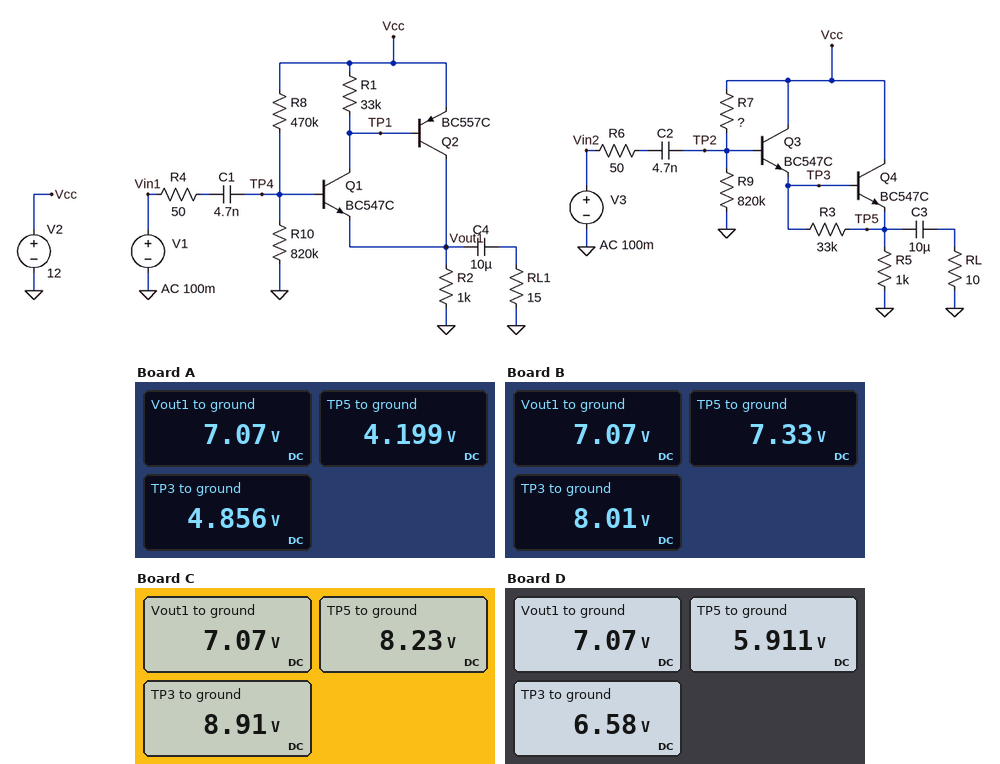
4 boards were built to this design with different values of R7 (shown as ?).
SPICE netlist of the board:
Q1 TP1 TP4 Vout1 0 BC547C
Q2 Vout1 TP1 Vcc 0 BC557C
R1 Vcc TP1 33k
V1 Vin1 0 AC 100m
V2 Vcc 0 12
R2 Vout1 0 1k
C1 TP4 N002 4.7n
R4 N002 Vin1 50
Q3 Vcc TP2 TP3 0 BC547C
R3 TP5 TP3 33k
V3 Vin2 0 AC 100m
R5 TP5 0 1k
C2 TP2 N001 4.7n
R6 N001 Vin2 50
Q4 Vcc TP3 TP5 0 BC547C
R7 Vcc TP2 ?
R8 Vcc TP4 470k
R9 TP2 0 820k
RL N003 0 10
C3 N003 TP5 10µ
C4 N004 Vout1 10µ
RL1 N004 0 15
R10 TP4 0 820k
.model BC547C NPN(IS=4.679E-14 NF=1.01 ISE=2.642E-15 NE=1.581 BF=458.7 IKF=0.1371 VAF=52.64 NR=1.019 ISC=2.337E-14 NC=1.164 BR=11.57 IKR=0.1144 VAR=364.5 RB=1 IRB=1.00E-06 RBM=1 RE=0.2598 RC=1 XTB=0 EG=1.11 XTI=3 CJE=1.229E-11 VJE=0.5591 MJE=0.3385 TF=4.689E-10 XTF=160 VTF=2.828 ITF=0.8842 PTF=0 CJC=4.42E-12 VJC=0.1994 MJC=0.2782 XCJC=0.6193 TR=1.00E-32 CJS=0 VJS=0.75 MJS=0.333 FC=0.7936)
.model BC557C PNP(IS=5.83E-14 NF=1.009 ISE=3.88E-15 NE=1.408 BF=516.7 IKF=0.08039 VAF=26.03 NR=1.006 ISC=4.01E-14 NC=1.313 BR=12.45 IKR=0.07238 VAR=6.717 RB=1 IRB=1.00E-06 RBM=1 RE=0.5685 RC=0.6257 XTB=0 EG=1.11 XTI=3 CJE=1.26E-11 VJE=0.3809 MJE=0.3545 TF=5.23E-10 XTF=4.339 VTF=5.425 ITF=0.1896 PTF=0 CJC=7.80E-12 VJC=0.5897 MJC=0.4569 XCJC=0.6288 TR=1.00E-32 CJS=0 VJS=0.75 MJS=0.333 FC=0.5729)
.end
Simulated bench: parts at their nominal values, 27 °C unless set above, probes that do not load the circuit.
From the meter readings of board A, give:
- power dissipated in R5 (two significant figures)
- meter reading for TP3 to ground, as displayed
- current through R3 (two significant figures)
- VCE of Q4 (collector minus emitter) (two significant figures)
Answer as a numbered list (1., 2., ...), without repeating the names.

1. 18 mW
2. 4.856 V
3. 20 µA
4. 7.8 V
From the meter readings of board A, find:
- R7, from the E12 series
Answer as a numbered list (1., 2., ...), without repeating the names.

1. 1 MΩ
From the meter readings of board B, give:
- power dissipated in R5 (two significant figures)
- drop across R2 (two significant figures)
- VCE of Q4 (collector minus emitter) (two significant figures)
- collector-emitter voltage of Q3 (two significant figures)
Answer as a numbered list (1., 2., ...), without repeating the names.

1. 54 mW
2. 7.1 V
3. 4.7 V
4. 4.0 V
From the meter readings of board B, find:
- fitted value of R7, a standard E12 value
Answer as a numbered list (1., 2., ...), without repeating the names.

1. 330 kΩ
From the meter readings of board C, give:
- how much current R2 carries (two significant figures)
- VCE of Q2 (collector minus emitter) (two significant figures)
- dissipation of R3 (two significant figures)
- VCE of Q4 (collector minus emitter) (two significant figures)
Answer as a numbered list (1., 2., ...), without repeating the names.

1. 7.1 mA
2. -4.9 V
3. 14 µW
4. 3.8 V
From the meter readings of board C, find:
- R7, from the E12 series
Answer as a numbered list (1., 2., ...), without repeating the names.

1. 220 kΩ
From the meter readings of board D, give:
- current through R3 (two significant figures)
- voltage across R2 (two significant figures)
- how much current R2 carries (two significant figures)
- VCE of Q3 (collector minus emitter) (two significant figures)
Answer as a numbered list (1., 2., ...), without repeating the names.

1. 20 µA
2. 7.1 V
3. 7.1 mA
4. 5.4 V
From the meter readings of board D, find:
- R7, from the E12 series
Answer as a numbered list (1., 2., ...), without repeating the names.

1. 560 kΩ
